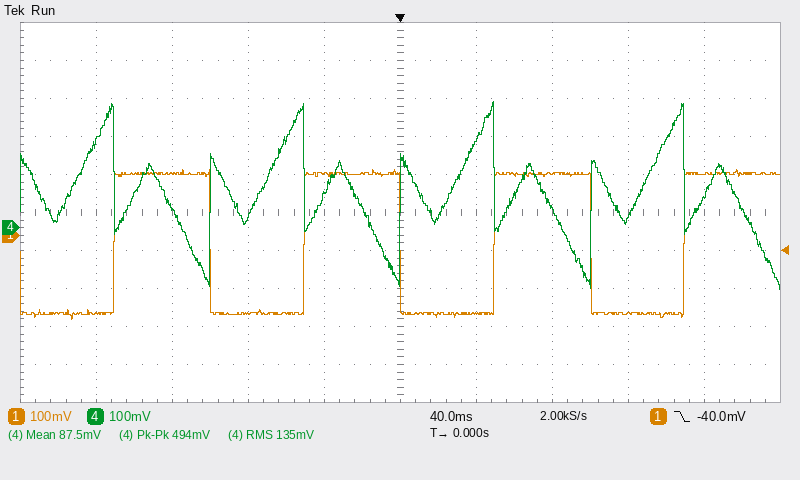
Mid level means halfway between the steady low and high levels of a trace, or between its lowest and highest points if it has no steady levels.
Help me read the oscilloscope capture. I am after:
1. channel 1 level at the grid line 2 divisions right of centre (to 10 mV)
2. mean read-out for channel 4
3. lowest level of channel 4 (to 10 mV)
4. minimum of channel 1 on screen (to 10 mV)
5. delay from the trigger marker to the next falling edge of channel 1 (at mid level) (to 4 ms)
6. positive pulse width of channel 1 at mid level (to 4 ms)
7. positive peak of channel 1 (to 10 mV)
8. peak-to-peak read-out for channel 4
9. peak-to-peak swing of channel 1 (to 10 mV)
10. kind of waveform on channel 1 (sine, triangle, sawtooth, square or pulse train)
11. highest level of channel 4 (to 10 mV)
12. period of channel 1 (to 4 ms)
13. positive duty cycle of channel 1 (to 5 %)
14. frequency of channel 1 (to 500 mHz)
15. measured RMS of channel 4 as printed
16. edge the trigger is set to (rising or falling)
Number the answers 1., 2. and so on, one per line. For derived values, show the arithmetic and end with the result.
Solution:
1. 160 mV
2. 87.5 mV
3. -160 mV
4. -220 mV
5. 100 ms
6. 52 ms
7. 170 mV
8. 494 mV
9. 170 mV − (-220 mV) = 390 mV
10. square
11. 330 mV
12. 100 ms
13. 52 ms / 100 ms ≈ 52.0 %, so 50 % to the nearest 5 %
14. 1 / 100 ms ≈ 10.0 Hz
15. 135 mV
16. falling
